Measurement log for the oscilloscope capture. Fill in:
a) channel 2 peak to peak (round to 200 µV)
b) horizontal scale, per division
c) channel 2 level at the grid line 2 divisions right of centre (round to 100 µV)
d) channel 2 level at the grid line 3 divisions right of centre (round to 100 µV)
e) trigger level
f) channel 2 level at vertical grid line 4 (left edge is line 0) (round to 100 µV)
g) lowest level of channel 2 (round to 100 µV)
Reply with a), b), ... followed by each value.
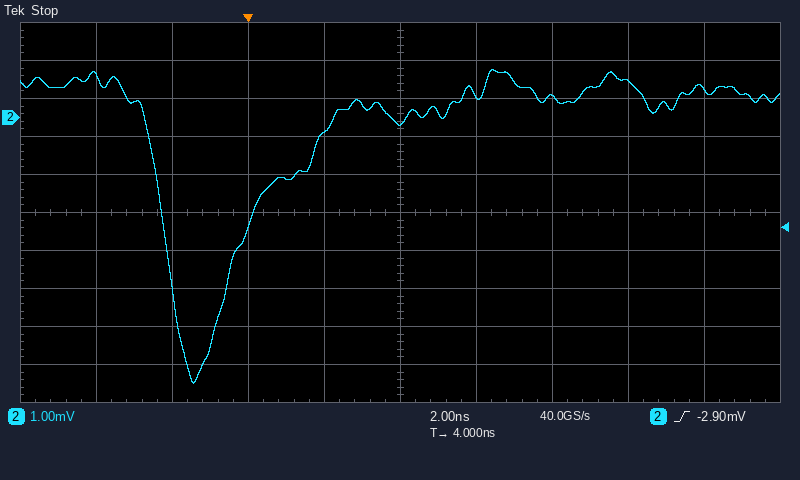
a) 8.2 mV
b) 2 ns
c) 500 µV
d) 900 µV
e) -2.90 mV
f) -400 µV
g) -7.0 mV
